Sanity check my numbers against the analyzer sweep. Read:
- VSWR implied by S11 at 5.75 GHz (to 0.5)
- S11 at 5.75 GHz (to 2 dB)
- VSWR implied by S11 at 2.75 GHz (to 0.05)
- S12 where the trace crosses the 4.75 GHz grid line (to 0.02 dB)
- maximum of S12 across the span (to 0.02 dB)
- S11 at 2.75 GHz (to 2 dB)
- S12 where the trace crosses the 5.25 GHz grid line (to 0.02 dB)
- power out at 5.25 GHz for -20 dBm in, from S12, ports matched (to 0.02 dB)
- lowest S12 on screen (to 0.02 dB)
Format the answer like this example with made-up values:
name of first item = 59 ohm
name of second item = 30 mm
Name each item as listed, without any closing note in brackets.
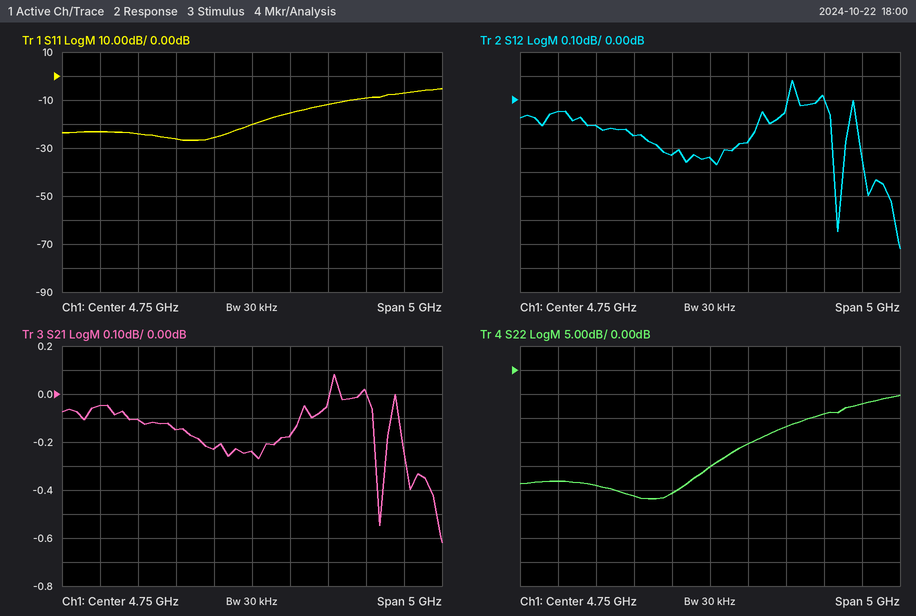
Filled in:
VSWR implied by S11 at 5.75 GHz = 1.5
S11 at 5.75 GHz = -12 dB
VSWR implied by S11 at 2.75 GHz = 1.15
S12 where the trace crosses the 4.75 GHz grid line = -0.24 dB
maximum of S12 across the span = 0.08 dB
S11 at 2.75 GHz = -24 dB
S12 where the trace crosses the 5.25 GHz grid line = -0.18 dB
power out at 5.25 GHz for -20 dBm in, from S12, ports matched = -20.18 dBm
lowest S12 on screen = -0.62 dB
